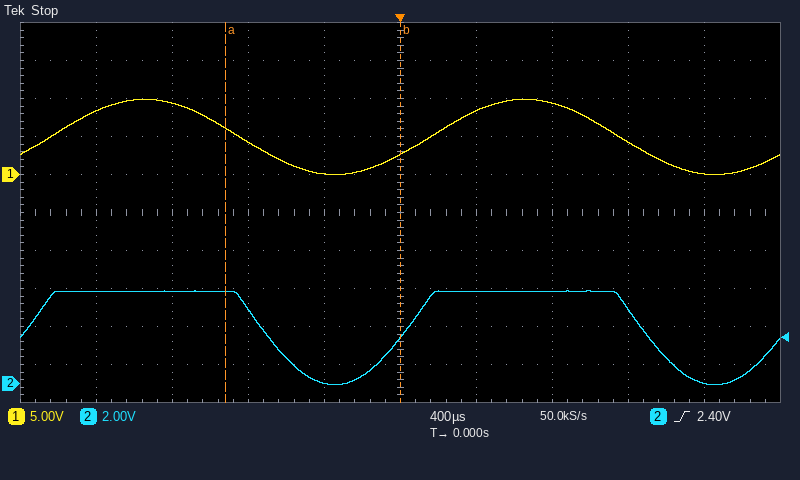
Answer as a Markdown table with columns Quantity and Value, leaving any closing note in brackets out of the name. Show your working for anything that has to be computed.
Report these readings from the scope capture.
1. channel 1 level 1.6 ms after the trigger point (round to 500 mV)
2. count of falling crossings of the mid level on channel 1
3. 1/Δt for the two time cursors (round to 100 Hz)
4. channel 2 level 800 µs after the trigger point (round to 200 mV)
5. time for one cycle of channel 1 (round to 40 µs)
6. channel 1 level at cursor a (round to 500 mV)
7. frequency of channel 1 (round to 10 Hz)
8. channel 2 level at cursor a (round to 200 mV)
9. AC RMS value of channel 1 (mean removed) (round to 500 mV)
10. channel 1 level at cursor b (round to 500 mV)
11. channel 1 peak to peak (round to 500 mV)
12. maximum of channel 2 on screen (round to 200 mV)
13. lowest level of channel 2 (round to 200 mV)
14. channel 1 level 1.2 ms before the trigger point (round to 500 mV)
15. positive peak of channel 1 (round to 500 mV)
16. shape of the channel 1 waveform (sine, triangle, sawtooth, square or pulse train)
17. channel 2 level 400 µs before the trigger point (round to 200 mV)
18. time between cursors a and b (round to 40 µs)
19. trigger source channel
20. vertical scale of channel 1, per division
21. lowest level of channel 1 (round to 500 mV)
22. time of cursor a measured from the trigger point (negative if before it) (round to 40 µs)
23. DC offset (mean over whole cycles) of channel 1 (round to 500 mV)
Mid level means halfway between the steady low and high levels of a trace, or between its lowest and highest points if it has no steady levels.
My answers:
| Quantity | Value |
|---|---|
| channel 1 level 1.6 ms after the trigger point | 0.0 V |
| count of falling crossings of the mid level on channel 1 | 2 |
| 1/Δt for the two time cursors | 1 / 920 µs ≈ 1.1 kHz |
| channel 2 level 800 µs after the trigger point | 4.8 V |
| time for one cycle of channel 1 | 2.00 ms |
| channel 1 level at cursor a | 6.0 V |
| frequency of channel 1 | 1 / 2.00 ms ≈ 500 Hz |
| channel 2 level at cursor a | 4.8 V |
| AC RMS value of channel 1 (mean removed) | 10.0 V / (2√2) ≈ 3.5 V |
| channel 1 level at cursor b | 2.5 V |
| channel 1 peak to peak | 10.0 V − (0.0 V) = 10.0 V |
| maximum of channel 2 on screen | 4.8 V |
| lowest level of channel 2 | 0.0 V |
| channel 1 level 1.2 ms before the trigger point | 9.5 V |
| positive peak of channel 1 | 10.0 V |
| shape of the channel 1 waveform | sine |
| channel 2 level 400 µs before the trigger point | 0.0 V |
| time between cursors a and b | 920 µs |
| trigger source channel | channel 2 |
| vertical scale of channel 1, per division | 5 V |
| lowest level of channel 1 | 0.0 V |
| time of cursor a measured from the trigger point (negative if before it) | -920 µs |
| DC offset (mean over whole cycles) of channel 1 | (10.0 V + (0.0 V)) / 2 ≈ 5.0 V |
